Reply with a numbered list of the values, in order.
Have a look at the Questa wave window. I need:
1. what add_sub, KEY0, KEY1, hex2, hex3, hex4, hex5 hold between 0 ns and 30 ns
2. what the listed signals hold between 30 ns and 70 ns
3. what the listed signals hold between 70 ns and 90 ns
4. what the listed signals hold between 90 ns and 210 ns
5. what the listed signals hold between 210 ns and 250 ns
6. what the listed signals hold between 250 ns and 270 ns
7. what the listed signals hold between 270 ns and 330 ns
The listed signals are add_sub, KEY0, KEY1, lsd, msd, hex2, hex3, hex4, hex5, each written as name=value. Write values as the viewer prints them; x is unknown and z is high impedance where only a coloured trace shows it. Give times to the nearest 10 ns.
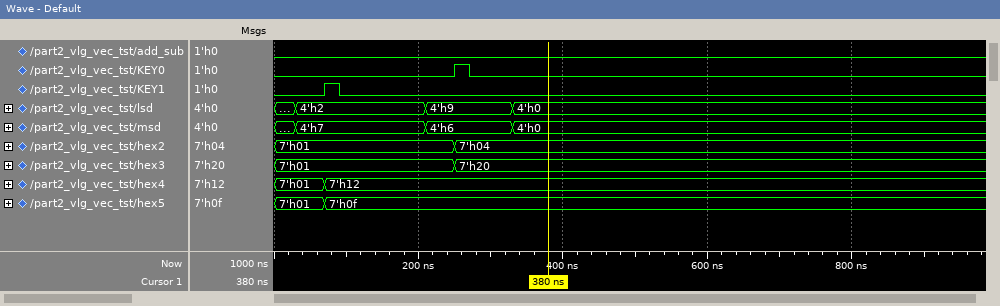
1. add_sub=0, KEY0=0, KEY1=0, hex2=7'h01, hex3=7'h01, hex4=7'h01, hex5=7'h01
2. add_sub=0, KEY0=0, KEY1=0, lsd=4'h2, msd=4'h7, hex2=7'h01, hex3=7'h01, hex4=7'h01, hex5=7'h01
3. add_sub=0, KEY0=0, KEY1=1, lsd=4'h2, msd=4'h7, hex2=7'h01, hex3=7'h01, hex4=7'h12, hex5=7'h0f
4. add_sub=0, KEY0=0, KEY1=0, lsd=4'h2, msd=4'h7, hex2=7'h01, hex3=7'h01, hex4=7'h12, hex5=7'h0f
5. add_sub=0, KEY0=0, KEY1=0, lsd=4'h9, msd=4'h6, hex2=7'h01, hex3=7'h01, hex4=7'h12, hex5=7'h0f
6. add_sub=0, KEY0=1, KEY1=0, lsd=4'h9, msd=4'h6, hex2=7'h04, hex3=7'h20, hex4=7'h12, hex5=7'h0f
7. add_sub=0, KEY0=0, KEY1=0, lsd=4'h9, msd=4'h6, hex2=7'h04, hex3=7'h20, hex4=7'h12, hex5=7'h0f
